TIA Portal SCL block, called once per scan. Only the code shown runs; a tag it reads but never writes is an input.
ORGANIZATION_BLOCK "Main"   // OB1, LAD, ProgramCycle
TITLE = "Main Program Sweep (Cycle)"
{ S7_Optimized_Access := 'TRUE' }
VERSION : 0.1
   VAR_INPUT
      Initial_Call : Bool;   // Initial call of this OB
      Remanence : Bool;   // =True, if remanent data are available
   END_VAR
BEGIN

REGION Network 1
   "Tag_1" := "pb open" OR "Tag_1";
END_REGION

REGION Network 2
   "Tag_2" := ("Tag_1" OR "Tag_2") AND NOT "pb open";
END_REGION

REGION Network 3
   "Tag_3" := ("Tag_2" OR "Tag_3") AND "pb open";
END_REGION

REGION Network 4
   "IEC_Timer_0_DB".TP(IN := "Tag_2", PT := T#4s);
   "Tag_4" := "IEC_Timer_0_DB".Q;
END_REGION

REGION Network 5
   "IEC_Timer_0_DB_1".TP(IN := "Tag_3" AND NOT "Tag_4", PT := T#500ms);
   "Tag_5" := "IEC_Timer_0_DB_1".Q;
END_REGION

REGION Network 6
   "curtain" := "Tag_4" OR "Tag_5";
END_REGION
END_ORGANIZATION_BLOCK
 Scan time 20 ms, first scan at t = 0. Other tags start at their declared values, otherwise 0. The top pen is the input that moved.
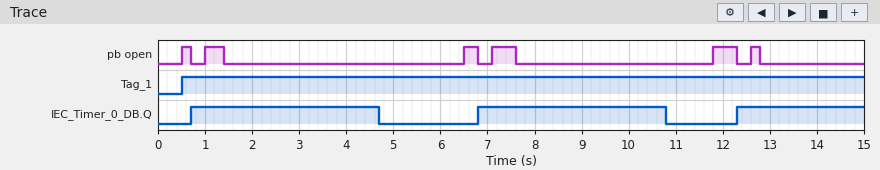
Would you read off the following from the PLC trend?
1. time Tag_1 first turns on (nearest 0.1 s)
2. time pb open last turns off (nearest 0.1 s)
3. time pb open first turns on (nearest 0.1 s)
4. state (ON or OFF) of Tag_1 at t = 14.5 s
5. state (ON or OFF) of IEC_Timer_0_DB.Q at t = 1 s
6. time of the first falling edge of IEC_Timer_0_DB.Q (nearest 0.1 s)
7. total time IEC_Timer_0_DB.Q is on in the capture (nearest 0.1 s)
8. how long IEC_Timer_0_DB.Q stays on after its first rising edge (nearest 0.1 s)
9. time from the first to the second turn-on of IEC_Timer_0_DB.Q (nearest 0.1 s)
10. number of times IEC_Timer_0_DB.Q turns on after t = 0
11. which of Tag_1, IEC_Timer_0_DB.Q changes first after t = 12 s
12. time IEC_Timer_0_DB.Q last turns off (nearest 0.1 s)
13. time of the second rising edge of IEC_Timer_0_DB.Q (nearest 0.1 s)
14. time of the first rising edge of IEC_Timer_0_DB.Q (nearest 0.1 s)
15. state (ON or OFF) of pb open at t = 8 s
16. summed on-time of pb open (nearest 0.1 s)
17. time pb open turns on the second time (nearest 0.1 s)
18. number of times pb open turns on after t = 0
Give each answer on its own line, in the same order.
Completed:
0.5 s
12.8 s
0.5 s
ON
ON
4.7 s
10.7 s
4.0 s
6.1 s
3
IEC_Timer_0_DB.Q
10.8 s
6.8 s
0.7 s
OFF
2.1 s
1.0 s
6
